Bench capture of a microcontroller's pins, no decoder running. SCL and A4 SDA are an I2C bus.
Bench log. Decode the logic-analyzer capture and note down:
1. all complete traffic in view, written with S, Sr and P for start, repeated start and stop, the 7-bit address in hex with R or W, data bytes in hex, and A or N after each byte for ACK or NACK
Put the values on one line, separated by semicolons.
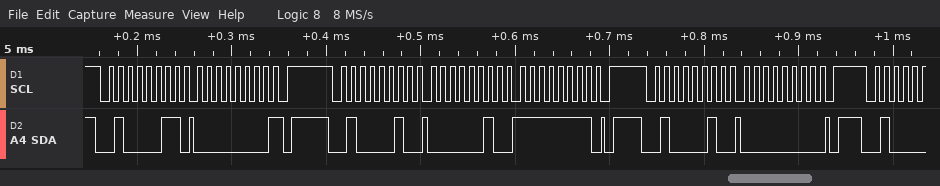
S 21R A 00 N P S 21W A 02 A FF A P S 21W A 00 A P
